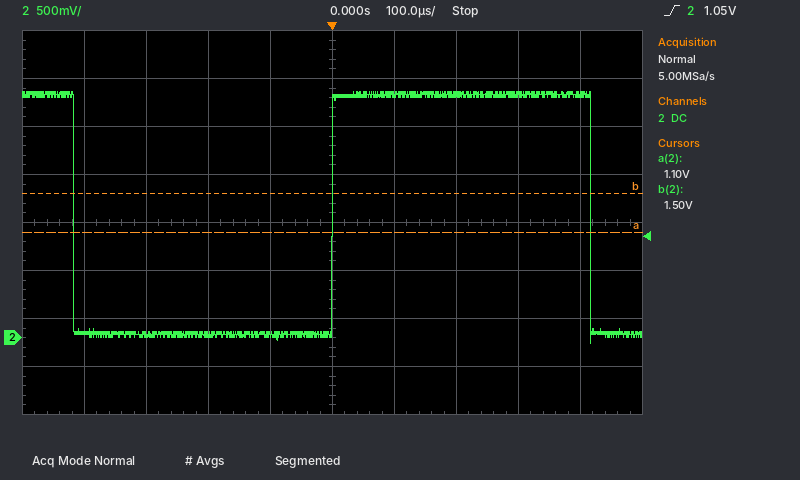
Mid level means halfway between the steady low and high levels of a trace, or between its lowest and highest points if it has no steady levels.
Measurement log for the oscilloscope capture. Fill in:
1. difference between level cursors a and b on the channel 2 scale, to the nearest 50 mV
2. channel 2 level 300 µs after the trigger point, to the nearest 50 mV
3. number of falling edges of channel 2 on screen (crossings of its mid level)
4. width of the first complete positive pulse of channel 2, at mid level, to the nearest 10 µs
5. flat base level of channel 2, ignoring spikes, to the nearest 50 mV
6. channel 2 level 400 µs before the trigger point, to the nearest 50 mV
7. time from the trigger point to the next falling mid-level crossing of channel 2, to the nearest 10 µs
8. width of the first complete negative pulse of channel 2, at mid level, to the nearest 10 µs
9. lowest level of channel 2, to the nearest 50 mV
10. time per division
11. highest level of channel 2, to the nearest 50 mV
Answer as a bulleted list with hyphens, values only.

- 400 mV
- 2.55 V
- 2
- 420 µs
- 50 mV
- 50 mV
- 420 µs
- 420 µs
- -50 mV
- 100 µs
- 2.55 V
